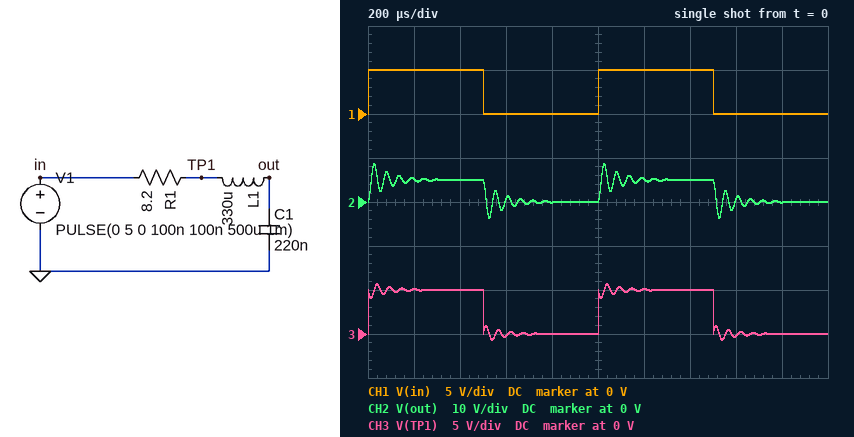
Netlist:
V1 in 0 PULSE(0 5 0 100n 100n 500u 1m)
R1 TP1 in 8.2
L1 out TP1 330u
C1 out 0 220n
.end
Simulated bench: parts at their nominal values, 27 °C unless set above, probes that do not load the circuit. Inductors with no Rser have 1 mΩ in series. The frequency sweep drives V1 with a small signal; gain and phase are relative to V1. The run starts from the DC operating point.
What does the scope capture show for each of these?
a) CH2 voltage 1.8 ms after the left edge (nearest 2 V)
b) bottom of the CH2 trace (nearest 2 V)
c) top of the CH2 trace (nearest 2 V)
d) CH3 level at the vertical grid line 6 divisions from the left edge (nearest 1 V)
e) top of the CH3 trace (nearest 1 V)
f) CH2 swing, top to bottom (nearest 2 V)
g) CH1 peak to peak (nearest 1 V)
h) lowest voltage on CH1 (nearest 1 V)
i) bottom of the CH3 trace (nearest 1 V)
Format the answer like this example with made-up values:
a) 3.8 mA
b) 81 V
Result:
a) 0 V
b) -4 V
c) 8 V
d) 5 V
e) 6 V
f) 12 V
g) 5 V
h) 0 V
i) -1 V
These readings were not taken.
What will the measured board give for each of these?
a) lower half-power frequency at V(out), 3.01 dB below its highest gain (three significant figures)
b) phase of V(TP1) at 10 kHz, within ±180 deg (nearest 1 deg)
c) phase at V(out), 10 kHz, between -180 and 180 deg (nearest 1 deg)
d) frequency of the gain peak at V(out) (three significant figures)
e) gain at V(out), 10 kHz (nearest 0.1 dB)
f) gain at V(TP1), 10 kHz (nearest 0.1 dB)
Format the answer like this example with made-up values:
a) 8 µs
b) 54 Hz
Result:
a) 16.4 kHz
b) -9 deg
c) -9 deg
d) 18.5 kHz
e) 2.8 dB
f) -0.1 dB
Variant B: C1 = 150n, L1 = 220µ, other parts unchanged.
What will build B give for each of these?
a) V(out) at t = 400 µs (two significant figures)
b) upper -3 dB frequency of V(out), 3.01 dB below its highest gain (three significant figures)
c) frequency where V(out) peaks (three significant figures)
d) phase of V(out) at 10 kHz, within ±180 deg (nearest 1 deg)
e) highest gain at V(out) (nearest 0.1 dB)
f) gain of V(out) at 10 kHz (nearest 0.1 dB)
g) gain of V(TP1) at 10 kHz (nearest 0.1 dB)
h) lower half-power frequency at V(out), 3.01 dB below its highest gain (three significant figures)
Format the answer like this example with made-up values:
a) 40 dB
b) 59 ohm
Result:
a) 5.0 V
b) 30.2 kHz
c) 27.4 kHz
d) -5 deg
e) 13.4 dB
f) 1.2 dB
g) 0 dB
h) 24.2 kHz
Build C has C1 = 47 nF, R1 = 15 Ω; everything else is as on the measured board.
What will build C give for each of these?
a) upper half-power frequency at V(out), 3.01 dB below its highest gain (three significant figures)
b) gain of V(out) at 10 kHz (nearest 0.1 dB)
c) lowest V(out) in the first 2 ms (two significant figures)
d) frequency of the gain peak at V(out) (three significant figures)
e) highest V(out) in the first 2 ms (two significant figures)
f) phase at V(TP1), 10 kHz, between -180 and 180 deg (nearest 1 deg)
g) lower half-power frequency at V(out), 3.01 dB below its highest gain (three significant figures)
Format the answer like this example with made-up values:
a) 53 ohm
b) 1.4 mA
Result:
a) 43.6 kHz
b) 0.5 dB
c) -3.8 V
d) 40.1 kHz
e) 8.8 V
f) -3 deg
g) 36.3 kHz
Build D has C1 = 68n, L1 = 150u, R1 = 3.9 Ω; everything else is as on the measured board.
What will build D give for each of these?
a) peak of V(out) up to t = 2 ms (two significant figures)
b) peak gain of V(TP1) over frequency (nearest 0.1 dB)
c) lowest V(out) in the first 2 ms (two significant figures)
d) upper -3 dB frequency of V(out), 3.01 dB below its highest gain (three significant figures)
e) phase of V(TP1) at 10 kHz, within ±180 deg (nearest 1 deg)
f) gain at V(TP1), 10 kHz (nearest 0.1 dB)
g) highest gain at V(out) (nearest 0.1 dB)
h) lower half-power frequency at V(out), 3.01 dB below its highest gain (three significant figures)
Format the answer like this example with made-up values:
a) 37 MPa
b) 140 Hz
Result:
a) 9.4 V
b) 0 dB
c) -4.4 V
d) 51.8 kHz
e) -1 deg
f) 0 dB
g) 21.6 dB
h) 47.6 kHz
